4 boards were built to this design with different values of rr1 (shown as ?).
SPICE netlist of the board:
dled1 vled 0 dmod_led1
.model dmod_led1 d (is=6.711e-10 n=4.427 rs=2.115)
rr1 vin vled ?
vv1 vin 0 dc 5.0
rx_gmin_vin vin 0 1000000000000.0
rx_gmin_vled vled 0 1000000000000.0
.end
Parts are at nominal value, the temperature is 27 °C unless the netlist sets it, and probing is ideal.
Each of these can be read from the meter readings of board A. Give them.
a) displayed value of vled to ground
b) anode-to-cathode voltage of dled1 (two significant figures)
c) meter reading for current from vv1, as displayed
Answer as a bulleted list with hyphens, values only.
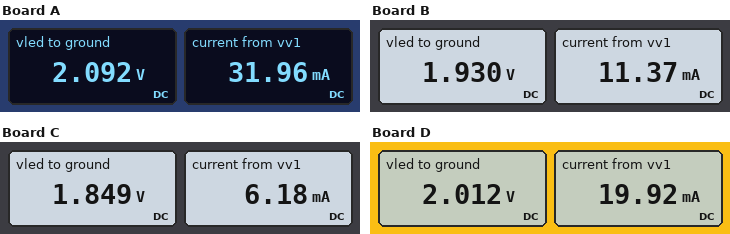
- 2.092 V
- 2.1 V
- 31.96 mA
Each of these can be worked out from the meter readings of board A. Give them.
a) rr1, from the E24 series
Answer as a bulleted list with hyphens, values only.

- 91 Ω
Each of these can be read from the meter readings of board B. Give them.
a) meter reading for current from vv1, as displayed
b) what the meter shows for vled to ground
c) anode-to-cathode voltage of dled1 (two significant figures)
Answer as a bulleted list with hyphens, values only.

- 11.37 mA
- 1.930 V
- 1.9 V
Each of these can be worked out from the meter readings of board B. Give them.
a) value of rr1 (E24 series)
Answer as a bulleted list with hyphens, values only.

- 270 Ω
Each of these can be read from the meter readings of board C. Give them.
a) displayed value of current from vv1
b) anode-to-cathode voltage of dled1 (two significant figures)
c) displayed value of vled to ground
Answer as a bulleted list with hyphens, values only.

- 6.18 mA
- 1.8 V
- 1.849 V
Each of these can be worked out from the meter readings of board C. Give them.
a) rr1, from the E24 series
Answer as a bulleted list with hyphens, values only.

- 510 Ω
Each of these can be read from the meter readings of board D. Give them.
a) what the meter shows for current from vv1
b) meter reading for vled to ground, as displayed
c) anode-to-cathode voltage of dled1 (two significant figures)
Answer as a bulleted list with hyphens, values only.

- 19.92 mA
- 2.012 V
- 2.0 V
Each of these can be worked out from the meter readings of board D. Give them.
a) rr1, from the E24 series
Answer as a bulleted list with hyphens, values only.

- 150 Ω
